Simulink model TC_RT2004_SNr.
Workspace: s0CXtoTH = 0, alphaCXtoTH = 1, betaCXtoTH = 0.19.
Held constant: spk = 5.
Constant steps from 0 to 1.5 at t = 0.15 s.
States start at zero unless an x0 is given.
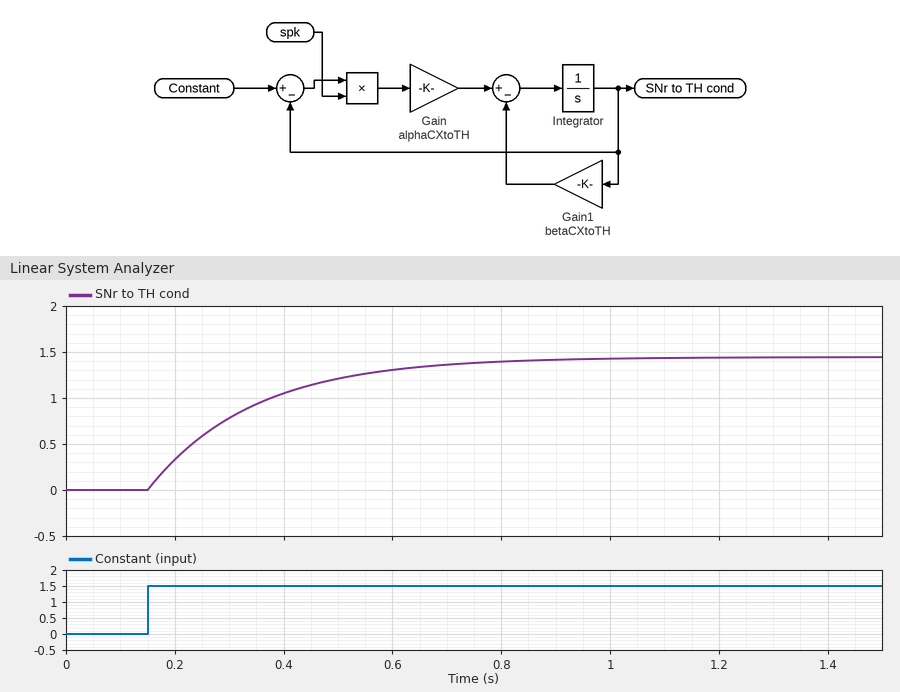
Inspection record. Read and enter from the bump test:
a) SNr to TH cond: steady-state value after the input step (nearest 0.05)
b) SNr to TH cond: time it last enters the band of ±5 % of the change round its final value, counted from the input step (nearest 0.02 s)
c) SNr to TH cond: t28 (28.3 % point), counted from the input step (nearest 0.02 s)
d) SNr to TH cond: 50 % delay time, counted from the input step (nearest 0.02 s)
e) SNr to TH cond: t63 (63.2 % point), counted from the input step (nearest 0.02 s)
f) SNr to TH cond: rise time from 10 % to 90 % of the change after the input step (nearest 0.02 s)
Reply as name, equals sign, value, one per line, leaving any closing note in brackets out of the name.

SNr to TH cond: steady-state value after the input step = 1.45
SNr to TH cond: time it last enters the band of ±5 % of the change round its final value, counted from the input step = 0.58 s
SNr to TH cond: t28 (28.3 % point), counted from the input step = 0.06 s
SNr to TH cond: 50 % delay time, counted from the input step = 0.14 s
SNr to TH cond: t63 (63.2 % point), counted from the input step = 0.20 s
SNr to TH cond: rise time from 10 % to 90 % of the change after the input step = 0.42 s
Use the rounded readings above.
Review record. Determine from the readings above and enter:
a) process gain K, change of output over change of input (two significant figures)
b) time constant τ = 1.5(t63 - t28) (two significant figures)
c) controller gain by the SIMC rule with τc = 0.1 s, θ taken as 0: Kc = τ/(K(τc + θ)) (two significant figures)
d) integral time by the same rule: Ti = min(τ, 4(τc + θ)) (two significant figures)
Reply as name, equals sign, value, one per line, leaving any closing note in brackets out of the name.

process gain K, change of output over change of input = 0.97
time constant τ = 1.5(t63 - t28) = 0.21 s
controller gain by the SIMC rule with τc = 0.1 s, θ taken as 0: Kc = τ/(K(τc + θ)) = 2.2
integral time by the same rule: Ti = min(τ, 4(τc + θ)) = 0.21 s
